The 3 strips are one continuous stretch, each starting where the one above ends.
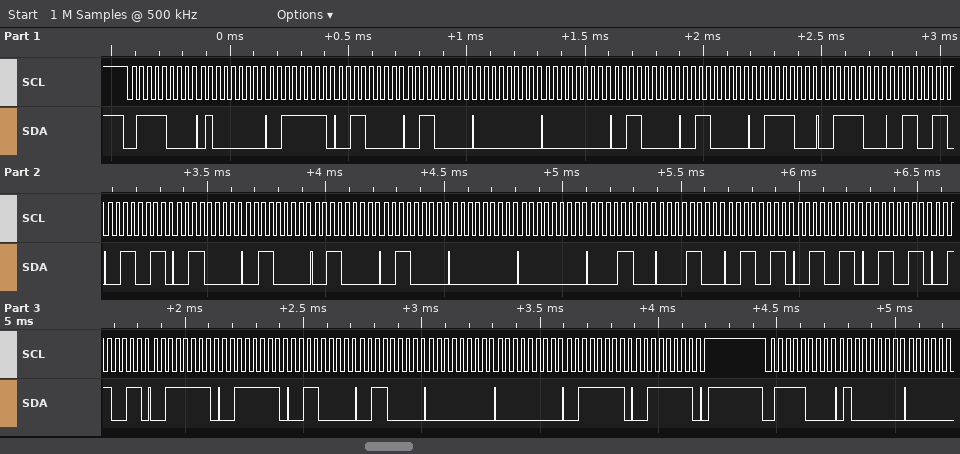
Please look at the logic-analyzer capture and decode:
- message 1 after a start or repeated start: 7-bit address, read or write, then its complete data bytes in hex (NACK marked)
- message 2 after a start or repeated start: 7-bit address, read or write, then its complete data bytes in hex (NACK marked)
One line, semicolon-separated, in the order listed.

0x3C write: 40 3F 30 30 00 00 30 30 3C 3C 33 33 30 30 30 30 00 00 0C 0C 33 33 33 33 3F 3F 30 30 00 00 3F 3F; 0x3C write: 40
